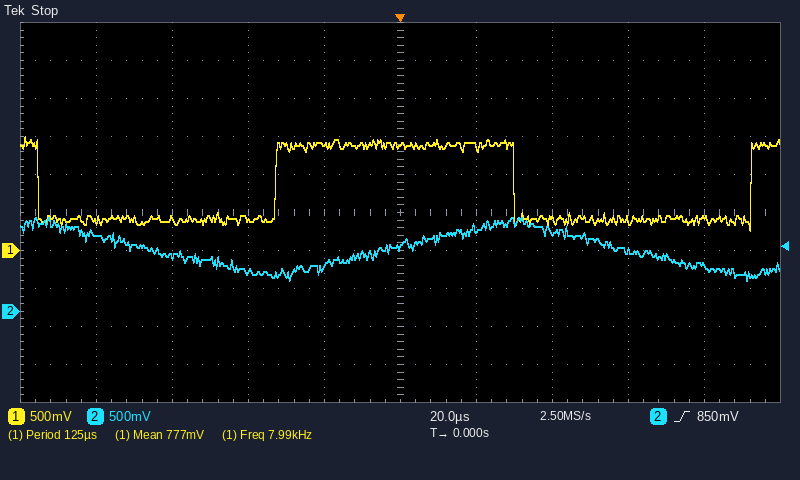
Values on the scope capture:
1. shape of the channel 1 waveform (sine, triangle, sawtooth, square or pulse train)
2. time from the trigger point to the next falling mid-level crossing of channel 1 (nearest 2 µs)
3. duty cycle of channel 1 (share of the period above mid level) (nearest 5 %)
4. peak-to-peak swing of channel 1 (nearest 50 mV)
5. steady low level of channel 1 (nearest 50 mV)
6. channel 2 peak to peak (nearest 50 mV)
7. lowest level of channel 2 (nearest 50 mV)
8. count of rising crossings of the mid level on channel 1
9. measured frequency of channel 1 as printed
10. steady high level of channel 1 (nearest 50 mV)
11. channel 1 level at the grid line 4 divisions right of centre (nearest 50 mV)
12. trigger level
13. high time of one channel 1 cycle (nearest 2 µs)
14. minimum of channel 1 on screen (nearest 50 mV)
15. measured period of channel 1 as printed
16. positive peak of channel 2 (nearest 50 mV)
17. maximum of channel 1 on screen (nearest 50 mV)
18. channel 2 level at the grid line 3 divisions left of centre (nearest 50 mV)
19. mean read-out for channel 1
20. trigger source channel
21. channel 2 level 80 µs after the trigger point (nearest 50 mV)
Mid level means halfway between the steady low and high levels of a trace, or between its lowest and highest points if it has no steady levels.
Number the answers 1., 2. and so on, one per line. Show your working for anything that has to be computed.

1. square
2. 30 µs
3. 50 %
4. 1.50 V − (250 mV) = 1.25 V
5. 400 mV
6. 1.25 V − (400 mV) = 850 mV
7. 400 mV
8. 2
9. 7.99 kHz
10. 1.40 V
11. 400 mV
12. 850 mV
13. 62 µs
14. 250 mV
15. 125 µs
16. 1.25 V
17. 1.50 V
18. 700 mV
19. 777 mV
20. channel 2
21. 600 mV
